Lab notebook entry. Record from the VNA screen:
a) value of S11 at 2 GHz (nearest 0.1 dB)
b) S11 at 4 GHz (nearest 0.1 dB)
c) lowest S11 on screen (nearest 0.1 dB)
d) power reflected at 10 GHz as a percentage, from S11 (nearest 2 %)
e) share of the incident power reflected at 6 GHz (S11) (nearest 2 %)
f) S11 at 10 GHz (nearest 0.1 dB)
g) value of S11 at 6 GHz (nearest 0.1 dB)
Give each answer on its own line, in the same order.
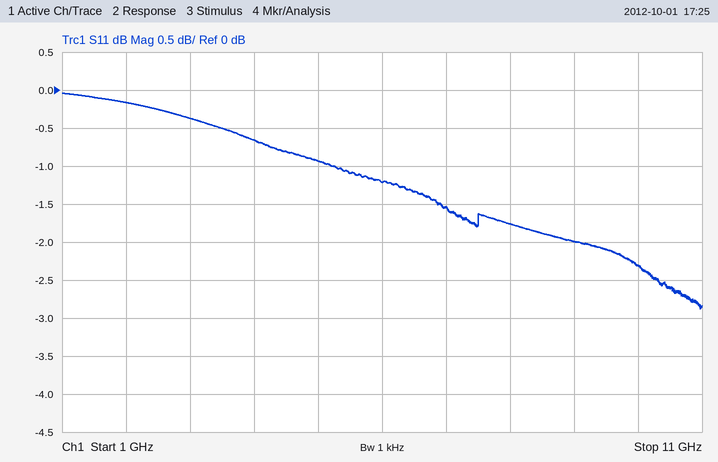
-0.2 dB
-0.7 dB
-2.9 dB
58 %
76 %
-2.3 dB
-1.2 dB
